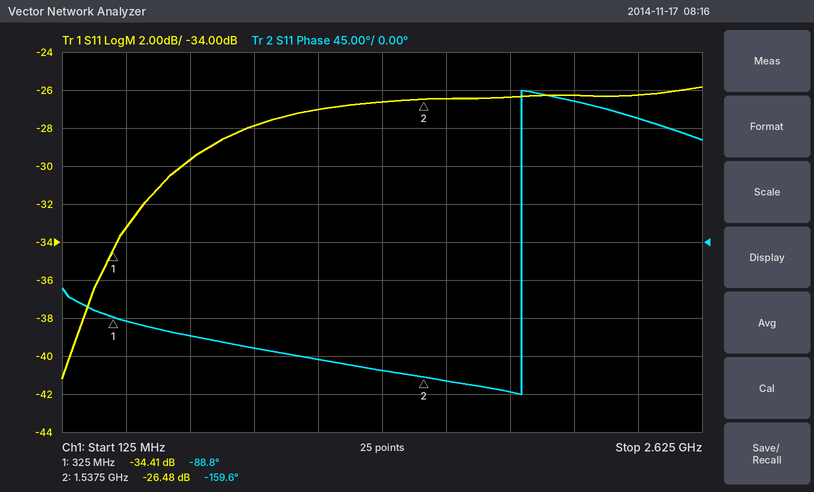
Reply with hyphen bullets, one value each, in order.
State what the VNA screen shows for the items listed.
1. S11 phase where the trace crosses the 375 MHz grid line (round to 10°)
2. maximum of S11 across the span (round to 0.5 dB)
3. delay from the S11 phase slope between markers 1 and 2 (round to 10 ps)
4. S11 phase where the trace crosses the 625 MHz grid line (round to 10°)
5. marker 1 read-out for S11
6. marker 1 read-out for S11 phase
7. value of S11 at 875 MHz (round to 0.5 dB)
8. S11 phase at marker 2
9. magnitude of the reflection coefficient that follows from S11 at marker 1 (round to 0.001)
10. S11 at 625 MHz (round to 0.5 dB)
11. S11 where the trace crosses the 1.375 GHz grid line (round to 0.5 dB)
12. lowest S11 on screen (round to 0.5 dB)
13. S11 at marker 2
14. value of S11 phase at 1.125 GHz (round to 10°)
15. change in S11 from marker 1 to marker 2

- -90°
- -26.0 dB
- 160 ps
- -110°
- -34.41 dB
- -88.8°
- -28.0 dB
- -159.6°
- 0.019
- -29.5 dB
- -26.5 dB
- -41.0 dB
- -26.48 dB
- -140°
- 7.93 dB
